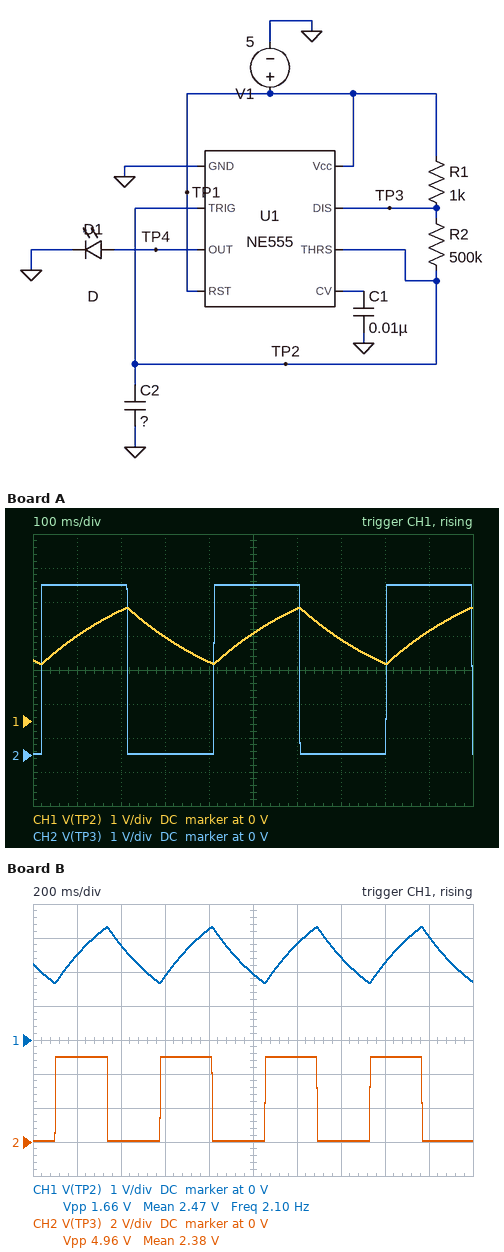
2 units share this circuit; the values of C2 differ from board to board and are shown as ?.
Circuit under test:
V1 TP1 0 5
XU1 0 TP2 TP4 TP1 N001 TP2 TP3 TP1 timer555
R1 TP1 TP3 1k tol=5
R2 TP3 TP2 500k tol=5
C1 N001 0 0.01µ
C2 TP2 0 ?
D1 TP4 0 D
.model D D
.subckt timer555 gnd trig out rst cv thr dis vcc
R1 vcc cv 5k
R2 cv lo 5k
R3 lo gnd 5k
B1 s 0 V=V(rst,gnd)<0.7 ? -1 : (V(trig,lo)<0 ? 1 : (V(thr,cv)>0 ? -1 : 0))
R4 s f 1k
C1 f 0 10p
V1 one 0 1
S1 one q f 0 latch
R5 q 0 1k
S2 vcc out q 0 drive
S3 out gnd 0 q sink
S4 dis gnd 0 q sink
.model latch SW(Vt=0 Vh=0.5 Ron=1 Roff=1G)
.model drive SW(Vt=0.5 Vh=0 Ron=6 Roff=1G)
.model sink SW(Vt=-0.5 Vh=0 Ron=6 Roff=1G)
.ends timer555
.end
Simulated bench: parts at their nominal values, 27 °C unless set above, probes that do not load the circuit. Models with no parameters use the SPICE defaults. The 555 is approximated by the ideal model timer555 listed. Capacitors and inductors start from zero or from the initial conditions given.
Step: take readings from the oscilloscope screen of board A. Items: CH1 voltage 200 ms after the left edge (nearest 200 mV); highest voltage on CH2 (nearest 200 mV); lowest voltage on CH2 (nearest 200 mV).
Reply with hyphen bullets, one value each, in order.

- 3.2 V
- 5.0 V
- 0 V
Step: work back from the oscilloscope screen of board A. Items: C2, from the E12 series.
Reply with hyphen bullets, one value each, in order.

- 560 nF
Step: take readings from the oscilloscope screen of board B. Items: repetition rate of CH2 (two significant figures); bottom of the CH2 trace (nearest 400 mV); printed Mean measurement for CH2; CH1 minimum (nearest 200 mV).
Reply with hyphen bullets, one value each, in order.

- 2.1 Hz
- 0 V
- 2.38 V
- 1.6 V
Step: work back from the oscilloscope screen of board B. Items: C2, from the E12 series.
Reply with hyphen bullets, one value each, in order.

- 680 nF
